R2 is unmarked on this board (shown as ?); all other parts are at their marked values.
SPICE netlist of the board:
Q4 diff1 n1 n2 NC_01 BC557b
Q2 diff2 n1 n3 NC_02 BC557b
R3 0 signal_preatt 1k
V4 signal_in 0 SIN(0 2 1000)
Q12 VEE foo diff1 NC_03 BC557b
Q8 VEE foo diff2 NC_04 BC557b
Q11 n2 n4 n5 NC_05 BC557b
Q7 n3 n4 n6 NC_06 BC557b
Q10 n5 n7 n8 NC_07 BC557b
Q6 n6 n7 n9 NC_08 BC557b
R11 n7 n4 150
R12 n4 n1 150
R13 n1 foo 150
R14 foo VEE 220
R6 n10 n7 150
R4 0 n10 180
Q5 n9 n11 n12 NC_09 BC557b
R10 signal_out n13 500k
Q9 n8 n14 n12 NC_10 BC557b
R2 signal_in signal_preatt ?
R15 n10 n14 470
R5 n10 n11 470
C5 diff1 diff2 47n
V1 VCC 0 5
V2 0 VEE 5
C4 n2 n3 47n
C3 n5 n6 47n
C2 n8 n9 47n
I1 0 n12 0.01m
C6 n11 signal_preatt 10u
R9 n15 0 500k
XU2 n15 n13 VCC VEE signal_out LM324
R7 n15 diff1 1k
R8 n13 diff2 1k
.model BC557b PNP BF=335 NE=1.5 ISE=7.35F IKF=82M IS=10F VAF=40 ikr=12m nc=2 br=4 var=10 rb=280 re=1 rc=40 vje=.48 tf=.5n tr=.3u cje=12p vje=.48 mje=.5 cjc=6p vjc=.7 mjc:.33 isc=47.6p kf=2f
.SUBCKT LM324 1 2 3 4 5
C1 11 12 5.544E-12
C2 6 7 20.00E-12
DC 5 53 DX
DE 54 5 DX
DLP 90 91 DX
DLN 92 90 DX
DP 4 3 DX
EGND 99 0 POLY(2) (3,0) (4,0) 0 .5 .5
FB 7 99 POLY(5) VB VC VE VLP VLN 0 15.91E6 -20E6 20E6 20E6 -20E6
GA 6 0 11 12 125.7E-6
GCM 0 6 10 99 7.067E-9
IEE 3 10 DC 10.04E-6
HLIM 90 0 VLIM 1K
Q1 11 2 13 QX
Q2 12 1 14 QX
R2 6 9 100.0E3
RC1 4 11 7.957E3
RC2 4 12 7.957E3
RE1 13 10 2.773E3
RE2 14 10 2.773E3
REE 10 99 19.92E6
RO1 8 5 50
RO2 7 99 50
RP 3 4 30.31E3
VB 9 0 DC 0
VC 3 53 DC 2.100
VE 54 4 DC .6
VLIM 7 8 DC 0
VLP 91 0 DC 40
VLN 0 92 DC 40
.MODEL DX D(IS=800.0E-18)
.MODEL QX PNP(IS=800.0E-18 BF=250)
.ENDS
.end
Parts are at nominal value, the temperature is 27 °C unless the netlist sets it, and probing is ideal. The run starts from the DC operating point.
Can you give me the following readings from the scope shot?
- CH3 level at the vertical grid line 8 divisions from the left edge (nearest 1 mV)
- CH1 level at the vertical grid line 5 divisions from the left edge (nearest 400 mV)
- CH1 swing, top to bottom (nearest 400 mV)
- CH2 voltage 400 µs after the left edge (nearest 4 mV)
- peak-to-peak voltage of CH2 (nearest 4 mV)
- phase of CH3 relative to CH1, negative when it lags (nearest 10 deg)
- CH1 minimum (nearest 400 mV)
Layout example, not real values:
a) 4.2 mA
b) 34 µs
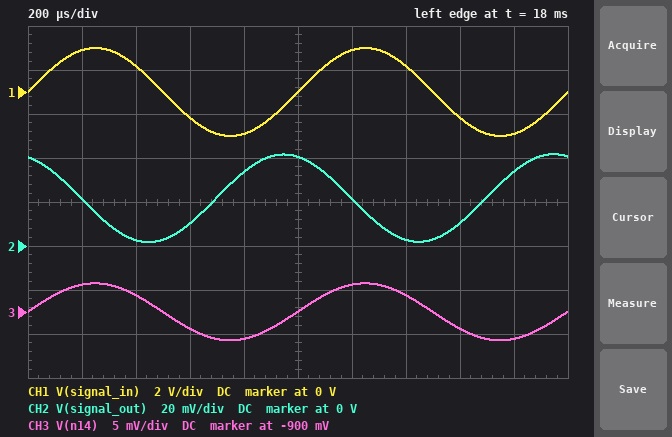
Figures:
a) -902 mV
b) 0 V
c) 4.0 V
d) 4 mV
e) 40 mV
f) 0 deg
g) -2.0 V
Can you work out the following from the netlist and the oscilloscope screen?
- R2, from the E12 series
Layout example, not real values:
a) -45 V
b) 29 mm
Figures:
a) 56 kΩ
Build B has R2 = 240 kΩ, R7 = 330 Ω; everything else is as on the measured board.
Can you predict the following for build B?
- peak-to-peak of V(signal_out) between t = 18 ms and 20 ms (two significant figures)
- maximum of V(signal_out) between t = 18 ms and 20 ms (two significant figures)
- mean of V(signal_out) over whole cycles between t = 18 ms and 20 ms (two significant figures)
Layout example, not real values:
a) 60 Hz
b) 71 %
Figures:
a) 9.3 mV
b) -640 mV
c) -650 mV
